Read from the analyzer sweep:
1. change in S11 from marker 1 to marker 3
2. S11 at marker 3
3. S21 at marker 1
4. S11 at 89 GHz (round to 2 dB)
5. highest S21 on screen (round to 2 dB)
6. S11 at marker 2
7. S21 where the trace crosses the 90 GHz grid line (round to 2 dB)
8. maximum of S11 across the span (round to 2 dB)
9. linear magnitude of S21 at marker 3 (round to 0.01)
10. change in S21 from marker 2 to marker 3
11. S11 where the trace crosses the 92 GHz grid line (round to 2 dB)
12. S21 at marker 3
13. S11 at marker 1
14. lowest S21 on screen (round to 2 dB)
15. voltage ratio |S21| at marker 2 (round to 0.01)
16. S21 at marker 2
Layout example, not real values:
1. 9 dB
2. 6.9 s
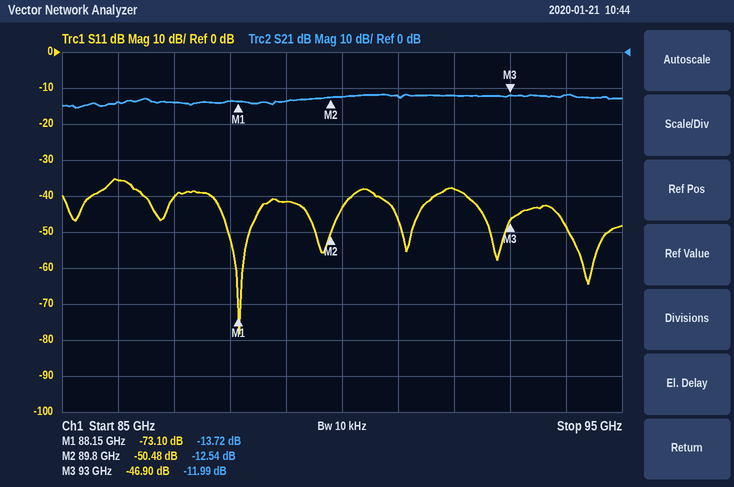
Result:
1. 26.20 dB
2. -46.90 dB
3. -13.72 dB
4. -42 dB
5. -12 dB
6. -50.48 dB
7. -12 dB
8. -36 dB
9. 0.25
10. 0.55 dB
11. -38 dB
12. -11.99 dB
13. -73.10 dB
14. -16 dB
15. 0.24
16. -12.54 dB
